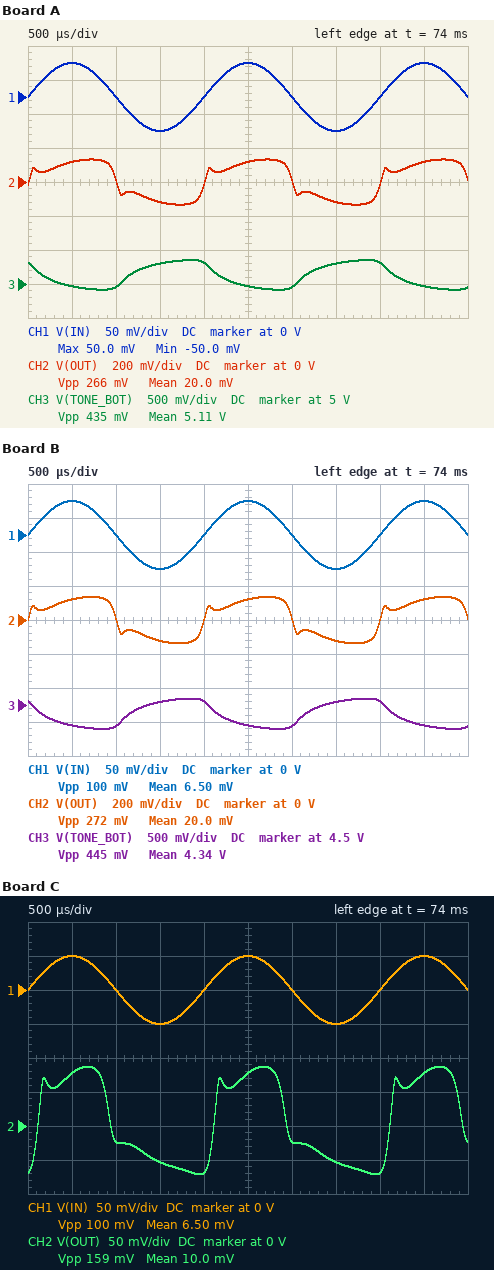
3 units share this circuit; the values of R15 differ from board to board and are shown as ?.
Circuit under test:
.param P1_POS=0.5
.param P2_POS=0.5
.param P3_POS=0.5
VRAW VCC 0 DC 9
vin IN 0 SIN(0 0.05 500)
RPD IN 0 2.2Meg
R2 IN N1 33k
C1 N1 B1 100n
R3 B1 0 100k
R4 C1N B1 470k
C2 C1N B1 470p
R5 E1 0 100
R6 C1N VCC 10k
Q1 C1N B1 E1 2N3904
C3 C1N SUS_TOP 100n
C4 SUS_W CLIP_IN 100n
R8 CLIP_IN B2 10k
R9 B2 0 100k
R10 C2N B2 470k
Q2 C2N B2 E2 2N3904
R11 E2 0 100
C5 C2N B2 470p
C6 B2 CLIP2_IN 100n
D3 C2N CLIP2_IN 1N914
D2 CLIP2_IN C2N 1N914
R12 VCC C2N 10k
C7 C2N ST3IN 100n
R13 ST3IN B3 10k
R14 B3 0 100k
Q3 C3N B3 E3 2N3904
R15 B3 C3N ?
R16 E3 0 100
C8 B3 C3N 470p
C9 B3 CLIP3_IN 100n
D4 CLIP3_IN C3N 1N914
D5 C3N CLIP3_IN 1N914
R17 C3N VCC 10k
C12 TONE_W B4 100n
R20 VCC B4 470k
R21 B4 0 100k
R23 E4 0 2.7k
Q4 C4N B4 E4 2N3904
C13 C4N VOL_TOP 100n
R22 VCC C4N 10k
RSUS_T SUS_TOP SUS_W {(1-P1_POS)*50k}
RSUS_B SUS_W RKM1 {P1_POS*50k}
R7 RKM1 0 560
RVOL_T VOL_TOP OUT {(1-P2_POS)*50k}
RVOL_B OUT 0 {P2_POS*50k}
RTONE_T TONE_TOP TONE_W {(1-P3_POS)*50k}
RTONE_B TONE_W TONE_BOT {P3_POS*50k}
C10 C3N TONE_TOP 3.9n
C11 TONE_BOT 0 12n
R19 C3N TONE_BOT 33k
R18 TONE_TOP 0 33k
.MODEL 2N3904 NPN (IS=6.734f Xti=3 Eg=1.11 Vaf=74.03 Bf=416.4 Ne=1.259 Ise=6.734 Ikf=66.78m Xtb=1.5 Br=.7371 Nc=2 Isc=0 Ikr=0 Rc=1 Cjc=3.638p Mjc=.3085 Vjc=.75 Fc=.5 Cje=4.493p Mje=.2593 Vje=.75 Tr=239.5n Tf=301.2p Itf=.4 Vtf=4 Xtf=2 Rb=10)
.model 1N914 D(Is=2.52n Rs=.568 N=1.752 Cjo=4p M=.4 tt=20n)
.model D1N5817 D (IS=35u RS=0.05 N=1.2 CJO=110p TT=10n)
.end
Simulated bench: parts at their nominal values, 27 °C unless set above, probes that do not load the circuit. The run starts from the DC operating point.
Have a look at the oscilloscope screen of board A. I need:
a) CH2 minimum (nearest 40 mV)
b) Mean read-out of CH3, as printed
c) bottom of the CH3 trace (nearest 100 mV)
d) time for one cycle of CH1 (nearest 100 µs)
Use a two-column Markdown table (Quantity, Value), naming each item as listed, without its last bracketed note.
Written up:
| Quantity | Value |
|---|---|
| CH2 minimum | -120 mV |
| Mean read-out of CH3, as printed | 5.11 V |
| bottom of the CH3 trace | 4.9 V |
| time for one cycle of CH1 | 2.0 ms |
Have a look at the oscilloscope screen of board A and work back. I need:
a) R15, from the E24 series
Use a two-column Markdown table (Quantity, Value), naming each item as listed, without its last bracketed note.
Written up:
| Quantity | Value |
|---|---|
| R15, from the E24 series | 560 kΩ |
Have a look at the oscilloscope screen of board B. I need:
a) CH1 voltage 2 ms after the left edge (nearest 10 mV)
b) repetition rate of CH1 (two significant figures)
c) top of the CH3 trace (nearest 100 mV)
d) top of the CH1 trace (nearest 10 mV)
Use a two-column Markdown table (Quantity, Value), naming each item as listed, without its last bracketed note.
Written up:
| Quantity | Value |
|---|---|
| CH1 voltage 2 ms after the left edge | 0 V |
| repetition rate of CH1 | 500 Hz |
| top of the CH3 trace | 4.6 V |
| top of the CH1 trace | 50 mV |
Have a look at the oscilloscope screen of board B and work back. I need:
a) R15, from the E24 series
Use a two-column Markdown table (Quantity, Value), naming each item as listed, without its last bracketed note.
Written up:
| Quantity | Value |
|---|---|
| R15, from the E24 series | 330 kΩ |
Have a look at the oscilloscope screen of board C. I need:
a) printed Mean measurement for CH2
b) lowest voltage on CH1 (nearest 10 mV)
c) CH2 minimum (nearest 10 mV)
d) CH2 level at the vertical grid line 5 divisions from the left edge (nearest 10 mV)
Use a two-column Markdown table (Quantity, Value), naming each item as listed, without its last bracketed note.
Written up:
| Quantity | Value |
|---|---|
| printed Mean measurement for CH2 | 10.0 mV |
| lowest voltage on CH1 | -50 mV |
| CH2 minimum | -70 mV |
| CH2 level at the vertical grid line 5 divisions from the left edge | 80 mV |
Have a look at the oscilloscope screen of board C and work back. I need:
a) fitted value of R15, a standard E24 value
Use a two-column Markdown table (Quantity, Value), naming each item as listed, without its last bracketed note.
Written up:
| Quantity | Value |
|---|---|
| fitted value of R15, a standard E24 value | 1.2 MΩ |
